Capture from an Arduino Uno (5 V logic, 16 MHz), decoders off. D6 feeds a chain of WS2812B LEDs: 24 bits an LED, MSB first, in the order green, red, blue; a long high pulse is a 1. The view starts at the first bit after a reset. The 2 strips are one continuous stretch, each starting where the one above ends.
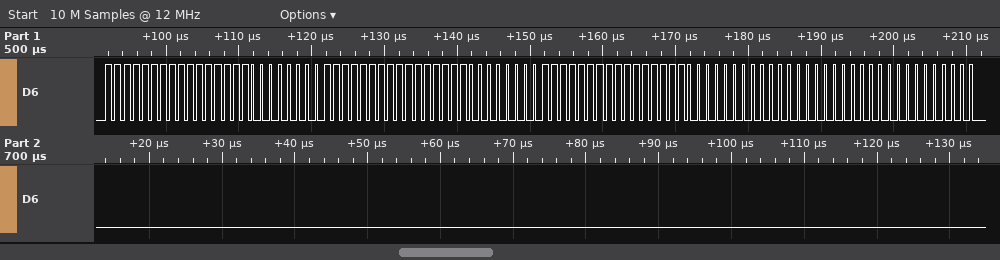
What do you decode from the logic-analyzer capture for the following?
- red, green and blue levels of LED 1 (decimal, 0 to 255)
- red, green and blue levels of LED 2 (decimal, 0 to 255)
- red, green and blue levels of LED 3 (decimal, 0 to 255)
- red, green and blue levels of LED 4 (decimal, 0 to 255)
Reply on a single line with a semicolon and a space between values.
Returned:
255, 255, 0; 255, 255, 0; 255, 255, 0; 0, 0, 0
